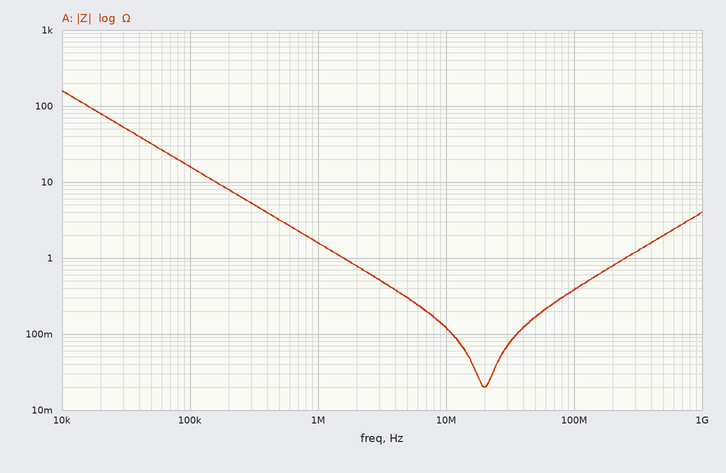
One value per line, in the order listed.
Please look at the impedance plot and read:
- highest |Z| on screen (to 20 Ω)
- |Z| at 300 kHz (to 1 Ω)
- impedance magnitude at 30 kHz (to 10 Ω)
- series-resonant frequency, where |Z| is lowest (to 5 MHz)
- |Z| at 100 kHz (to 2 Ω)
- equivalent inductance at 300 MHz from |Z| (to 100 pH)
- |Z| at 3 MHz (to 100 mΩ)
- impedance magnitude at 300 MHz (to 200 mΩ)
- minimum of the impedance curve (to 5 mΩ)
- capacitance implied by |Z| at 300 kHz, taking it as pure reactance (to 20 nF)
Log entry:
160 Ω
5 Ω
50 Ω
20 MHz
16 Ω
600 pH
500 mΩ
1.2 Ω
20 mΩ
100 nF
